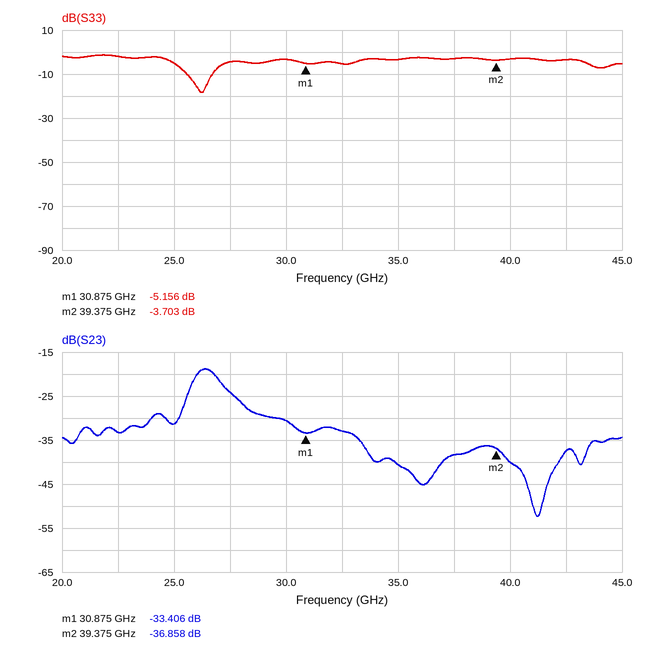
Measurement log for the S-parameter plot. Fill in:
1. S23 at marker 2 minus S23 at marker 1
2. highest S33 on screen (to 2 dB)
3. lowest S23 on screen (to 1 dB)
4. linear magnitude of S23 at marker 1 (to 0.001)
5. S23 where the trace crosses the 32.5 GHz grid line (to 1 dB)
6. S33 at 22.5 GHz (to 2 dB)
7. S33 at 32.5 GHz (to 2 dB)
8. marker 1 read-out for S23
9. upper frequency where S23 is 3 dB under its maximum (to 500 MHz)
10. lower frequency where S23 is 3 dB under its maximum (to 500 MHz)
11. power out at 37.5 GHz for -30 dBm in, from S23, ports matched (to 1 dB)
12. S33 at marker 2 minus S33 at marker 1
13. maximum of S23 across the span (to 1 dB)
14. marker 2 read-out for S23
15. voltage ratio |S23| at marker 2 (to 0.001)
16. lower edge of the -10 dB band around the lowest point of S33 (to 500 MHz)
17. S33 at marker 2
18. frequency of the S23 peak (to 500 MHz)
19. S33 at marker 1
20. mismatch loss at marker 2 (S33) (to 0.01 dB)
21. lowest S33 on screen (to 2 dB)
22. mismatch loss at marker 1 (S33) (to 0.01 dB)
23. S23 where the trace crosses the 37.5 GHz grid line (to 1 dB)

-3.452 dB
-2 dB
-52 dB
0.021
-33 dB
-2 dB
-6 dB
-33.406 dB
27.0 GHz
26.0 GHz
-68 dBm
1.453 dB
-19 dB
-36.858 dB
0.014
25.5 GHz
-3.703 dB
26.5 GHz
-5.156 dB
2.41 dB
-18 dB
1.58 dB
-38 dB
